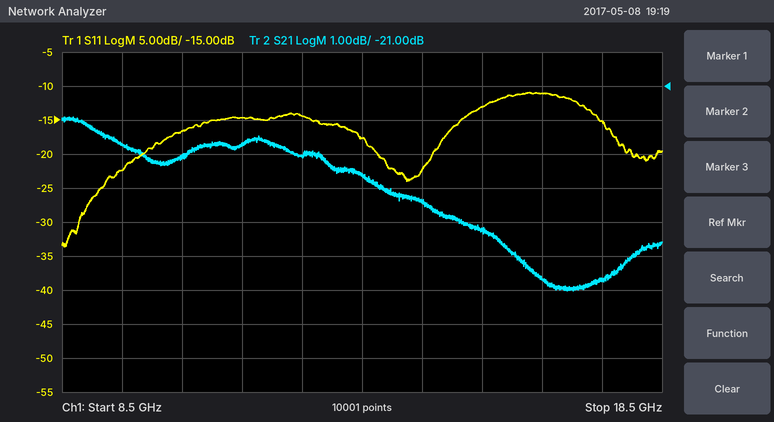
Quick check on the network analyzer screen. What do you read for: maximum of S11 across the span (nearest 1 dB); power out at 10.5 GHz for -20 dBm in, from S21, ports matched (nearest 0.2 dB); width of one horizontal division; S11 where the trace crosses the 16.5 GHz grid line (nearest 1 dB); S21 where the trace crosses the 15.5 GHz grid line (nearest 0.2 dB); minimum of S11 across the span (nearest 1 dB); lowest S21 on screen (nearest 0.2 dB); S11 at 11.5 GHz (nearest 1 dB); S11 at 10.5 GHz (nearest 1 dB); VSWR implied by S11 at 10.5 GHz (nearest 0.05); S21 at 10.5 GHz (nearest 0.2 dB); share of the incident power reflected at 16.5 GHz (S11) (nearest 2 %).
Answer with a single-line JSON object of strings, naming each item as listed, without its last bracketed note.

{"maximum of S11 across the span": "-11 dB", "power out at 10.5 GHz for -20 dBm in, from S21, ports matched": "-43.0 dBm", "width of one horizontal division": "1 GHz", "S11 where the trace crosses the 16.5 GHz grid line": "-11 dB", "S21 where the trace crosses the 15.5 GHz grid line": "-25.2 dB", "minimum of S11 across the span": "-34 dB", "lowest S21 on screen": "-27.0 dB", "S11 at 11.5 GHz": "-15 dB", "S11 at 10.5 GHz": "-17 dB", "VSWR implied by S11 at 10.5 GHz": "1.35", "S21 at 10.5 GHz": "-23.0 dB", "share of the incident power reflected at 16.5 GHz (S11)": "8 %"}
